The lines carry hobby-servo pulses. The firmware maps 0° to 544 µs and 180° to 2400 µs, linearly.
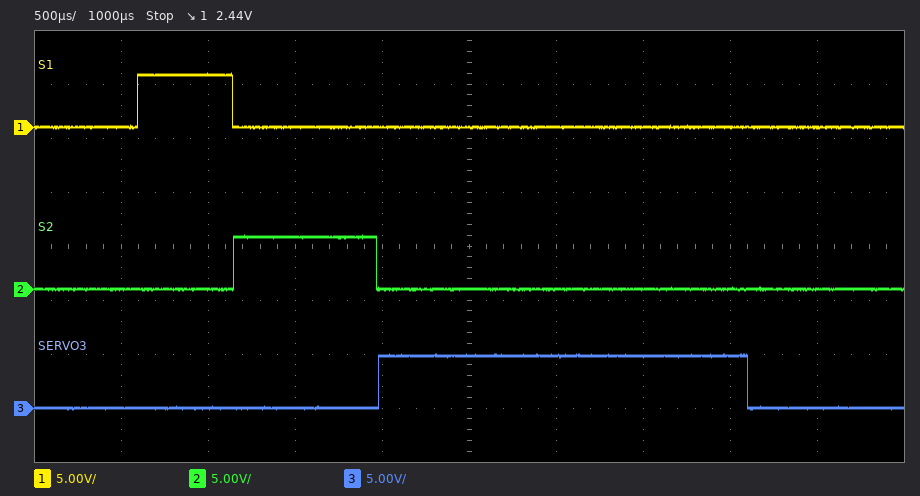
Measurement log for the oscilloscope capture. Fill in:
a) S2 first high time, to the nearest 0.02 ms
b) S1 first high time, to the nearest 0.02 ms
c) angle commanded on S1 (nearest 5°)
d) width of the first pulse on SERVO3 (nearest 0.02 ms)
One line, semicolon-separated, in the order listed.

0.82 ms; 0.54 ms; 0°; 2.12 ms
